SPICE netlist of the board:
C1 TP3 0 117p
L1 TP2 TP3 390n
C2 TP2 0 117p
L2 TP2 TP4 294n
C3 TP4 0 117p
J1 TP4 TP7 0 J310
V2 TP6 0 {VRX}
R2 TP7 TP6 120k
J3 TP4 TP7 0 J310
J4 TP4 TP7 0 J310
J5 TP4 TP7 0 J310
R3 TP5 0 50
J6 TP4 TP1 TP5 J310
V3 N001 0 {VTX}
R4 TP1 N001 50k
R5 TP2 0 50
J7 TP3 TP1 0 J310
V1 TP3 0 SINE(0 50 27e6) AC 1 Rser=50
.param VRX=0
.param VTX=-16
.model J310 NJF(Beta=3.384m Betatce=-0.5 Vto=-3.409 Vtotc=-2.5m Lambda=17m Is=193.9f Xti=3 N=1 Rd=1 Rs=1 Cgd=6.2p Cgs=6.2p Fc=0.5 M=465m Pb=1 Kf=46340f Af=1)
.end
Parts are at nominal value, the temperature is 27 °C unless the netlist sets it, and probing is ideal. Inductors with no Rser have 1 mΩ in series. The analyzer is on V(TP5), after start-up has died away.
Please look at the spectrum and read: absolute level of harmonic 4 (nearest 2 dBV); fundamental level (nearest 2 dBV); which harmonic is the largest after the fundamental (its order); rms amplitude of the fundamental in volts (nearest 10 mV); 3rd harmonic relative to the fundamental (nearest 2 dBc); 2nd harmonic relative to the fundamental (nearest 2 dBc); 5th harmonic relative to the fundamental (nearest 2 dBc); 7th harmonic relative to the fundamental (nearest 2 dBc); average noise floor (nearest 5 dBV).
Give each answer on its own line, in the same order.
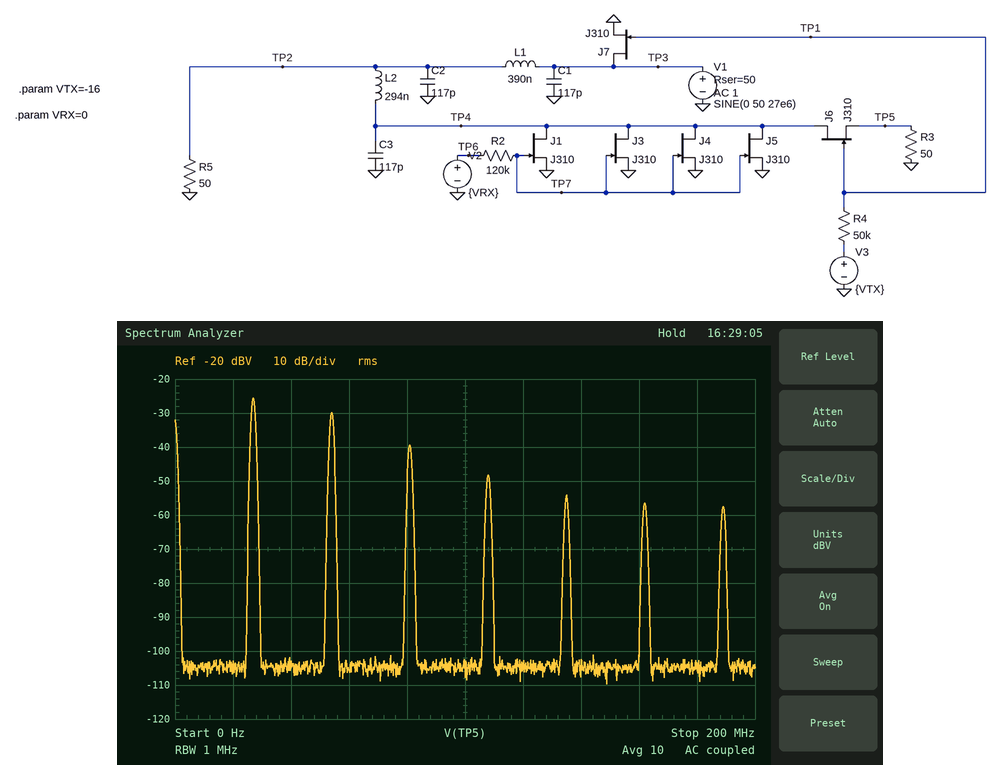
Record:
-48 dBV
-26 dBV
2
50 mV
-14 dBc
-4 dBc
-28 dBc
-32 dBc
-105 dBV
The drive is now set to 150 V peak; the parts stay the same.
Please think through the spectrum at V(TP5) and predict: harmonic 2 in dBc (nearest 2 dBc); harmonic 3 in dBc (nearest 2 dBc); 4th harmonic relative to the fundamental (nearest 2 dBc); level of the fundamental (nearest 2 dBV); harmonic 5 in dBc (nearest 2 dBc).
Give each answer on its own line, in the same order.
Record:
2 dBc
-10 dBc
-12 dBc
-22 dBV
-20 dBc
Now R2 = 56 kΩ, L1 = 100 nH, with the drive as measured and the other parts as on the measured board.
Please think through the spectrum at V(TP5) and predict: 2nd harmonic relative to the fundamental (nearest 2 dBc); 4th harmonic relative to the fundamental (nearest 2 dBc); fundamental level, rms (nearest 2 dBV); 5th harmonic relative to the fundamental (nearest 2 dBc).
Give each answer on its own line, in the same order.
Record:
-2 dBc
-10 dBc
-2 dBV
-20 dBc
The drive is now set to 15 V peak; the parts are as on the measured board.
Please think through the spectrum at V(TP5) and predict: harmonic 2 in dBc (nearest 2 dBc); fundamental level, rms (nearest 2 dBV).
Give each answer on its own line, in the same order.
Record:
-20 dBc
-34 dBV
